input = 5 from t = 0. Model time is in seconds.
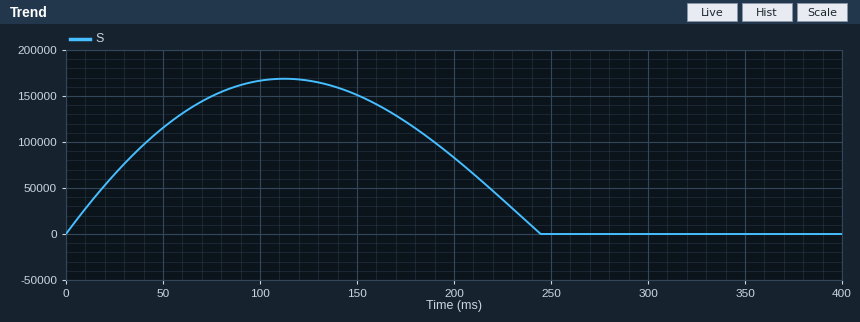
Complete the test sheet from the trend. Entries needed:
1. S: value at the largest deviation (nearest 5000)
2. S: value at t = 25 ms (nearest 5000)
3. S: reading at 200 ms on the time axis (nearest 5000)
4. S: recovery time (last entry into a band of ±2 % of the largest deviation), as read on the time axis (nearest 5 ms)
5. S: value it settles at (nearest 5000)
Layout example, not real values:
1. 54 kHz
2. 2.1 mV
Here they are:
1. 170000
2. 65000
3. 85000
4. 245 ms
5. 0
